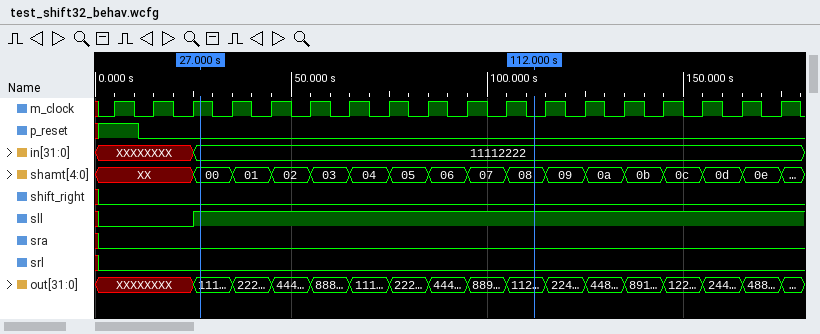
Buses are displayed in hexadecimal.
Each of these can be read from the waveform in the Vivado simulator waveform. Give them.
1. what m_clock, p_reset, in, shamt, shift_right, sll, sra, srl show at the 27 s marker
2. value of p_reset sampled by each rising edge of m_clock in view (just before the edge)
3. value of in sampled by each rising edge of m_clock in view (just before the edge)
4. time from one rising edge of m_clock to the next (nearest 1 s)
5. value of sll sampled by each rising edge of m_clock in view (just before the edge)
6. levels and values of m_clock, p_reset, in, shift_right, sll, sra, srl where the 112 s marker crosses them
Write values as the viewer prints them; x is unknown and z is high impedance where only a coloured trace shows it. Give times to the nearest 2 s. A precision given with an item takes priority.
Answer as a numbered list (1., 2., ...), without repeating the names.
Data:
1. m_clock=1, p_reset=0, in=11112222, shamt=00, shift_right=0, sll=1, sra=0, srl=0
2. 1 0 0 0 0 0 0 0 0 0 0 0 0 0 0 0 0 0
3. XXXXXXXX, XXXXXXXX, XXXXXXXX, 11112222, 11112222, 11112222, 11112222, 11112222, 11112222, 11112222, 11112222, 11112222, 11112222, 11112222, 11112222, 11112222, 11112222, 11112222
4. 10 s
5. 0 0 0 1 1 1 1 1 1 1 1 1 1 1 1 1 1 1
6. m_clock=0, p_reset=0, in=11112222, shift_right=0, sll=1, sra=0, srl=0
